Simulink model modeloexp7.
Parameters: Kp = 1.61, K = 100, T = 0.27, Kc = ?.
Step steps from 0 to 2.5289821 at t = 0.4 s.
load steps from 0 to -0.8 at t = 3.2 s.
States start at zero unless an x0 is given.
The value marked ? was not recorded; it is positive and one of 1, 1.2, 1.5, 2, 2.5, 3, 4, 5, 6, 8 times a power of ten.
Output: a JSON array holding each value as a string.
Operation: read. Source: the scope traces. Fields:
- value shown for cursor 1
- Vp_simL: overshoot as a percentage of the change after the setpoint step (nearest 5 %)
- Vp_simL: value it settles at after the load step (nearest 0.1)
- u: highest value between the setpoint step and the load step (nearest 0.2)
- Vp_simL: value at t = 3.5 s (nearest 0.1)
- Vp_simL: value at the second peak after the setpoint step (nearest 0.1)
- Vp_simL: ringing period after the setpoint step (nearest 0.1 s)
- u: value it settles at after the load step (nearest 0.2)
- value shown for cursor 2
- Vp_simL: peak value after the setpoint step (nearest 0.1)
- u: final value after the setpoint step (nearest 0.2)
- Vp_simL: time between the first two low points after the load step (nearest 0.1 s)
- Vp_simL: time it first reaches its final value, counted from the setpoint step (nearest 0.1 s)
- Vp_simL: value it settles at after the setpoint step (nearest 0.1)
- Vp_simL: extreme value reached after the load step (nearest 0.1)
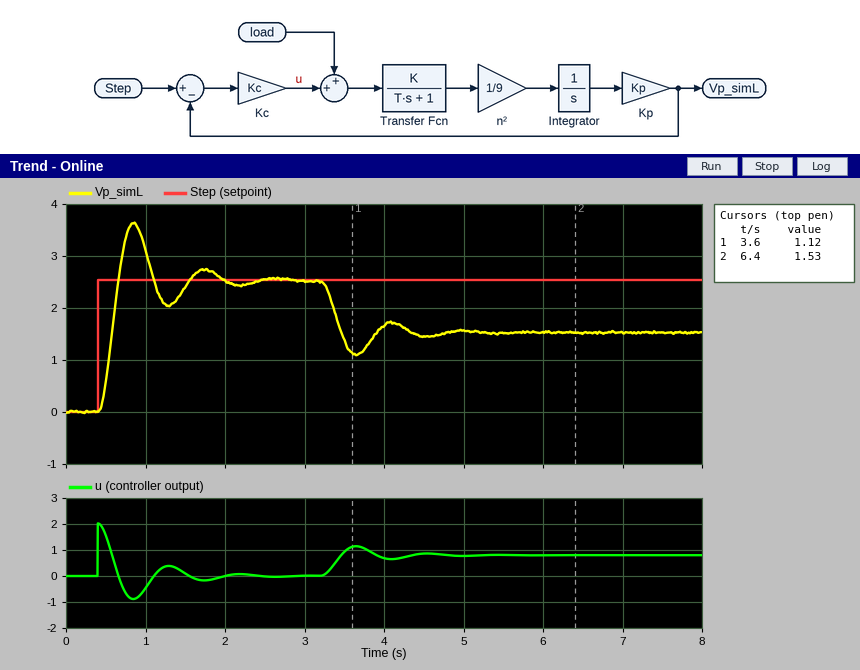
["1.12", "45 %", "1.5", "2.0", "1.4", "2.7", "0.9 s", "0.8", "1.53", "3.6", "0.0", "0.9 s", "0.3 s", "2.5", "1.1"]
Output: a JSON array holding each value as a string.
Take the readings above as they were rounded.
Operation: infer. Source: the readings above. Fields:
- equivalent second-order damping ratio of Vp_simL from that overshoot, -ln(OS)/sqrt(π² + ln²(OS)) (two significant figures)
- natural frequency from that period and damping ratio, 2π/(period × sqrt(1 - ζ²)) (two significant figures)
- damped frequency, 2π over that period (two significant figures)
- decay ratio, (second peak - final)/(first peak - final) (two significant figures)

["0.25", "7.2 rad/s", "7.0 rad/s", "0.18"]
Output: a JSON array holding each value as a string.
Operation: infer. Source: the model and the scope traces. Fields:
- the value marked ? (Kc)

["0.8"]
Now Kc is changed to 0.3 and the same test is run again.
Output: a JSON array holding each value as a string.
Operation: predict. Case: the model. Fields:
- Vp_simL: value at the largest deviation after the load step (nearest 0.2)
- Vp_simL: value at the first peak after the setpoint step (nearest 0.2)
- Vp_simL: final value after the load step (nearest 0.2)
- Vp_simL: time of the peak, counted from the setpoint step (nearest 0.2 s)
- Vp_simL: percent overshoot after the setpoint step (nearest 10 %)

["-0.8", "3.2", "-0.2", "0.8 s", "20 %"]
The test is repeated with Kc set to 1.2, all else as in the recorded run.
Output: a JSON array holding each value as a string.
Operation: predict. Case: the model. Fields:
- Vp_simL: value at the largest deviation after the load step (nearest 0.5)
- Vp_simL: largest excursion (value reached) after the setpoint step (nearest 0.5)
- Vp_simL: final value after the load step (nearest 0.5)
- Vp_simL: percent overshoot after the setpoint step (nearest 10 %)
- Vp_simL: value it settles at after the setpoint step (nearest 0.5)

["1.5", "4.0", "2.0", "50 %", "2.5"]
